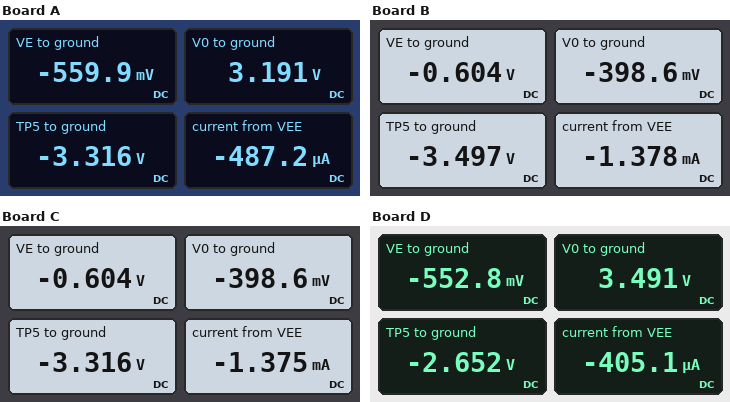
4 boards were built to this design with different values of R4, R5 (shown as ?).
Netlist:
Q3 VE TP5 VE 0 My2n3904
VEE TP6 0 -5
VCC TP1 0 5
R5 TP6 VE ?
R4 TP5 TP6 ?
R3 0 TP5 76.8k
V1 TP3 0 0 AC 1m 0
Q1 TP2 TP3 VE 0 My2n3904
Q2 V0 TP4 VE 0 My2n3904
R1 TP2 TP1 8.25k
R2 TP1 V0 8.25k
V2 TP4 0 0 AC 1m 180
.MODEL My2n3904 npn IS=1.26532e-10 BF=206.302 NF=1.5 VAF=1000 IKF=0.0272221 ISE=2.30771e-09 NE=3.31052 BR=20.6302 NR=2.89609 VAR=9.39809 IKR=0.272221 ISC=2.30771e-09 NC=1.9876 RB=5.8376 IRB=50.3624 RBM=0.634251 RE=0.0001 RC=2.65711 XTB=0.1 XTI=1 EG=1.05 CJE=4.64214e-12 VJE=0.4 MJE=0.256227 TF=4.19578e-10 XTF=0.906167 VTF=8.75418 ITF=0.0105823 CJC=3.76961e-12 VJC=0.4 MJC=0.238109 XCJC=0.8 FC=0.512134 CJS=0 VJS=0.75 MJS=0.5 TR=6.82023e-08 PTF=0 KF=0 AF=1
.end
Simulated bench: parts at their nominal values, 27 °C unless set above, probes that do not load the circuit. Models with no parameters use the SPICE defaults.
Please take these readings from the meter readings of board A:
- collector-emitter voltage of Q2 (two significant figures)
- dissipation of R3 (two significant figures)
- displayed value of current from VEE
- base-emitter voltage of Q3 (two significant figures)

3.8 V
140 µW
-487.2 µA
-2.8 V
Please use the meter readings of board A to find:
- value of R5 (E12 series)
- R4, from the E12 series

10 kΩ
39 kΩ
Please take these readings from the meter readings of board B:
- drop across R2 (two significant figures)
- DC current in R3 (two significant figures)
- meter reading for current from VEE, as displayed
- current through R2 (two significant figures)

5.4 V
46 µA
-1.378 mA
650 µA
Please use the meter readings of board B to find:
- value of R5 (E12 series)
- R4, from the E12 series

3.3 kΩ
33 kΩ
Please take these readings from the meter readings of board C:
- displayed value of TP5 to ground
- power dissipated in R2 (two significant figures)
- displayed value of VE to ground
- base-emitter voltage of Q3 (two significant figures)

-3.316 V
3.5 mW
-0.604 V
-2.7 V
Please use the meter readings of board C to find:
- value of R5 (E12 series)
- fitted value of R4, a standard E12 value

3.3 kΩ
39 kΩ
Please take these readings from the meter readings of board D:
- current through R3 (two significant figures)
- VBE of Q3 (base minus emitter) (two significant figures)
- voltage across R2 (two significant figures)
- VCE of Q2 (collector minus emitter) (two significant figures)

35 µA
-2.1 V
1.5 V
4.0 V
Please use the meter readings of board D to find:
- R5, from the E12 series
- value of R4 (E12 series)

12 kΩ
68 kΩ
